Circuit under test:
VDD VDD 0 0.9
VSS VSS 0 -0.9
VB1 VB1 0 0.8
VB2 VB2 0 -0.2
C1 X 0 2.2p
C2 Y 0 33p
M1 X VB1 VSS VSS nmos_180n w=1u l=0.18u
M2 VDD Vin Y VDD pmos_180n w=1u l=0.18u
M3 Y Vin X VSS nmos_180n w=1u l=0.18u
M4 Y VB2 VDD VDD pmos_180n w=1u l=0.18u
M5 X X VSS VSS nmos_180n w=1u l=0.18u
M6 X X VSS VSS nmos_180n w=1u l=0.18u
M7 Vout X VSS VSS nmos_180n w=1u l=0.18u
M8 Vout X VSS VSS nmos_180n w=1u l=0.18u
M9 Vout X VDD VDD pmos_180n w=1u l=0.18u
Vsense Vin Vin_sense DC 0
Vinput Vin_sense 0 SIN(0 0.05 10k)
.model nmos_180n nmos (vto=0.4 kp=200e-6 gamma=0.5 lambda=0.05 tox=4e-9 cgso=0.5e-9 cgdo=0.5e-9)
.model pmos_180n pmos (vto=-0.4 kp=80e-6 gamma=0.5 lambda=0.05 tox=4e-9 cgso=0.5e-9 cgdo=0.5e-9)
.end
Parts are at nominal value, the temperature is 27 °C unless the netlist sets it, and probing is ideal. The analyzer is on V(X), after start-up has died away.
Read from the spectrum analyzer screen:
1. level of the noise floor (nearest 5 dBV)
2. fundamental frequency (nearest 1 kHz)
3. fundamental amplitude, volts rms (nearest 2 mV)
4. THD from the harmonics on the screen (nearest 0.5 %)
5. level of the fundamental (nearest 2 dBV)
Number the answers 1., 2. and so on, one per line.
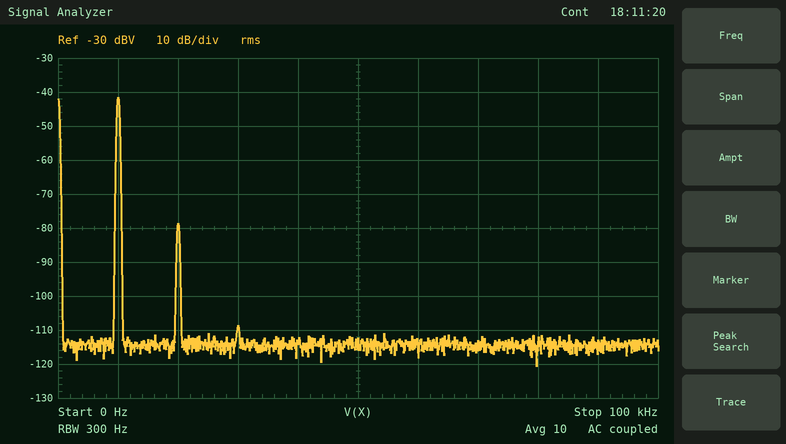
1. -115 dBV
2. 10 kHz
3. 8 mV
4. 1.5 %
5. -42 dBV
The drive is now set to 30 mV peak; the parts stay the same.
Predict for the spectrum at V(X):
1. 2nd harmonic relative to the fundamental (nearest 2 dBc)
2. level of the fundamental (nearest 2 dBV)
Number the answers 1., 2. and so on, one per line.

1. -42 dBc
2. -46 dBV
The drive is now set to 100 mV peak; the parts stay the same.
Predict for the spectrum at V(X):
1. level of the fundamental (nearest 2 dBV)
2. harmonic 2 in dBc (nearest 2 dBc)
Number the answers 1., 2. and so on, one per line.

1. -36 dBV
2. -32 dBc
